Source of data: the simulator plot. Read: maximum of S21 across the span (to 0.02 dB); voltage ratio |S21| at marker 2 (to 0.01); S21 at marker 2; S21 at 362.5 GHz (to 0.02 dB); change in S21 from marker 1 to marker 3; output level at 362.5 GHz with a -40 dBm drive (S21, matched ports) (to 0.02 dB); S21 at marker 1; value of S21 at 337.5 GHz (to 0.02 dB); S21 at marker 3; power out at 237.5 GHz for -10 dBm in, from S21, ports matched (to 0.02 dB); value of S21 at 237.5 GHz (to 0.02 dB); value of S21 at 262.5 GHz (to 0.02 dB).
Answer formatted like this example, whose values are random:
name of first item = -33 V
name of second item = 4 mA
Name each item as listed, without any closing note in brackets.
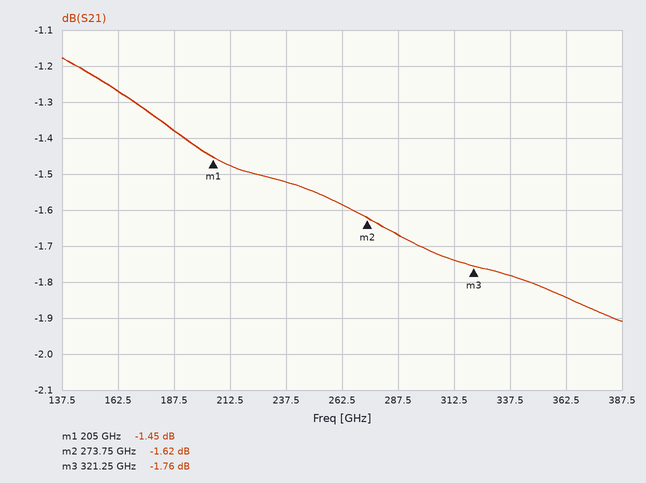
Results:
maximum of S21 across the span = -1.18 dB
voltage ratio |S21| at marker 2 = 0.83
S21 at marker 2 = -1.62 dB
S21 at 362.5 GHz = -1.84 dB
change in S21 from marker 1 to marker 3 = -0.31 dB
output level at 362.5 GHz with a -40 dBm drive (S21, matched ports) = -41.84 dBm
S21 at marker 1 = -1.45 dB
value of S21 at 337.5 GHz = -1.78 dB
S21 at marker 3 = -1.76 dB
power out at 237.5 GHz for -10 dBm in, from S21, ports matched = -11.52 dBm
value of S21 at 237.5 GHz = -1.52 dB
value of S21 at 262.5 GHz = -1.58 dB
